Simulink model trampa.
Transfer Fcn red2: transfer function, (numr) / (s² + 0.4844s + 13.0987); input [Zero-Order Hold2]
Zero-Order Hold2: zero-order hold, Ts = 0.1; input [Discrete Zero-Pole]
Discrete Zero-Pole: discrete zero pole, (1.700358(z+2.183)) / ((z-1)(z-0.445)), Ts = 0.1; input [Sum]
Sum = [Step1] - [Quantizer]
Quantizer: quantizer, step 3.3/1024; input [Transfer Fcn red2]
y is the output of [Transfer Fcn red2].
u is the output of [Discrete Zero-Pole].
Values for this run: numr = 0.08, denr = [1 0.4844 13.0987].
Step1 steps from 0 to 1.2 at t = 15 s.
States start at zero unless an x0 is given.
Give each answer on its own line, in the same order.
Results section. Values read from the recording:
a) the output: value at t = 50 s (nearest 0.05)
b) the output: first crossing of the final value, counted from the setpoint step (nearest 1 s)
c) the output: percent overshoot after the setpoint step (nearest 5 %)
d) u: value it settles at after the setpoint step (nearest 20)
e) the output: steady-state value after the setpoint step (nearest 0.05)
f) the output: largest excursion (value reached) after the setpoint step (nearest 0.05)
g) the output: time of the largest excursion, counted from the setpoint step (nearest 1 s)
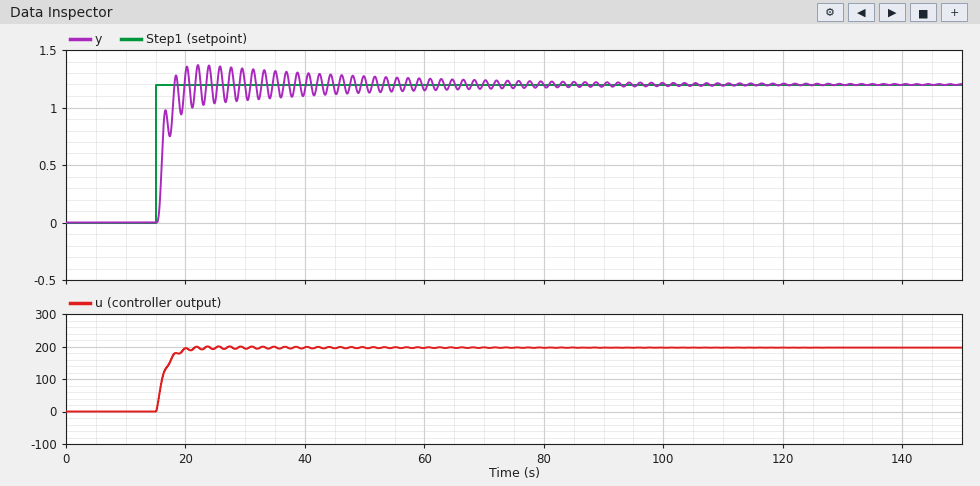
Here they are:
1.25
3 s
15 %
200
1.20
1.35
7 s
